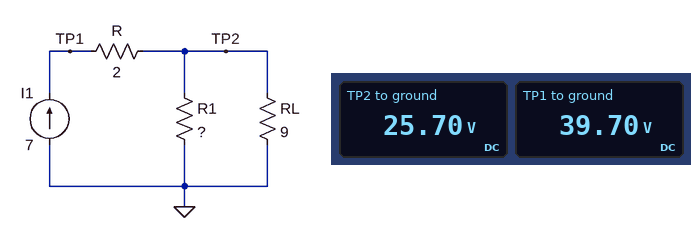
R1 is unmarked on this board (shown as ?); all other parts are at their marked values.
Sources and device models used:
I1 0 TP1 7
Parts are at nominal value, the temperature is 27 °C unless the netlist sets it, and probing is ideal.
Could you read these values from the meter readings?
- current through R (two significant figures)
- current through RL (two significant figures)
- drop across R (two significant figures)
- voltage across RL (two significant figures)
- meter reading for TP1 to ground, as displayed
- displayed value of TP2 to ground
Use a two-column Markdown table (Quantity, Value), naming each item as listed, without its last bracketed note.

| Quantity | Value |
|---|---|
| current through R | 7.0 A |
| current through RL | 2.9 A |
| drop across R | 14 V |
| voltage across RL | 26 V |
| meter reading for TP1 to ground, as displayed | 39.70 V |
| displayed value of TP2 to ground | 25.70 V |
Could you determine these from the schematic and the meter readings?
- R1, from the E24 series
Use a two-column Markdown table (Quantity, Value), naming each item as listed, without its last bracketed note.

| Quantity | Value |
|---|---|
| R1, from the E24 series | 6.2 Ω |
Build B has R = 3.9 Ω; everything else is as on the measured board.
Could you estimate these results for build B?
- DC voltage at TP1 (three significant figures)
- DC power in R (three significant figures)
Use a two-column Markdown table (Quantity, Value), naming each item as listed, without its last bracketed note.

| Quantity | Value |
|---|---|
| DC voltage at TP1 | 53.0 V |
| DC power in R | 191 W |
